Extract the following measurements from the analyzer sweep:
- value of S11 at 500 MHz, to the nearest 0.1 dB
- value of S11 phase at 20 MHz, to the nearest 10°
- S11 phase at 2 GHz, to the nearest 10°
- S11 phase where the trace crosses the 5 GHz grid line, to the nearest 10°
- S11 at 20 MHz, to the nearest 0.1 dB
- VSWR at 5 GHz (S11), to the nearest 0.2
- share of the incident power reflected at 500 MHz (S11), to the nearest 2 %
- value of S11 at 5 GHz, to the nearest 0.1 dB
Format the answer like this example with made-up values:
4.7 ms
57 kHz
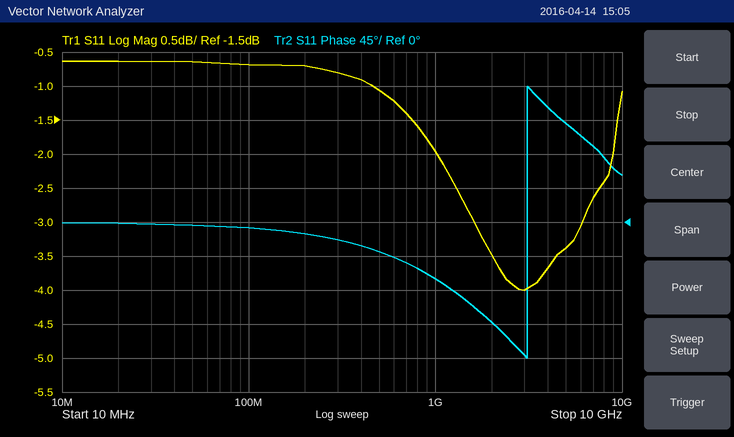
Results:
-1.1 dB
0°
-130°
130°
-0.6 dB
5.2
78 %
-3.4 dB
